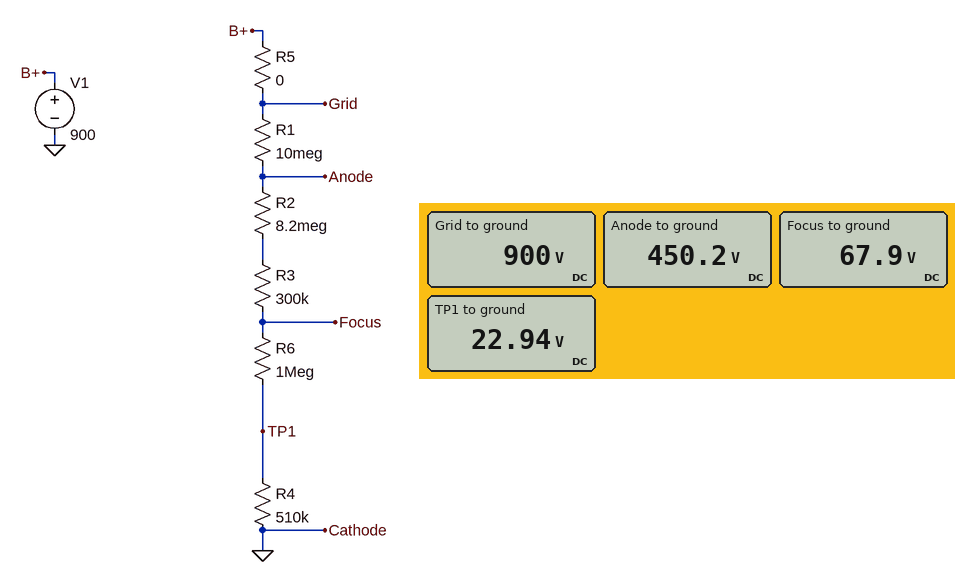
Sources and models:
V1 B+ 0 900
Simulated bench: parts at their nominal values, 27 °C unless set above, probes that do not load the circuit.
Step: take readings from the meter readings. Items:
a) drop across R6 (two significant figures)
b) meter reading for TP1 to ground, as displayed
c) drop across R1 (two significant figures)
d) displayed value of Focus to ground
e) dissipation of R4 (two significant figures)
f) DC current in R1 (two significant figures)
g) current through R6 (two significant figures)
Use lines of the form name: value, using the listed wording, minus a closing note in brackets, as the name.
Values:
drop across R6: 45 V
meter reading for TP1 to ground, as displayed: 22.94 V
drop across R1: 450 V
displayed value of Focus to ground: 67.9 V
dissipation of R4: 1.0 mW
DC current in R1: 45 µA
current through R6: 45 µA
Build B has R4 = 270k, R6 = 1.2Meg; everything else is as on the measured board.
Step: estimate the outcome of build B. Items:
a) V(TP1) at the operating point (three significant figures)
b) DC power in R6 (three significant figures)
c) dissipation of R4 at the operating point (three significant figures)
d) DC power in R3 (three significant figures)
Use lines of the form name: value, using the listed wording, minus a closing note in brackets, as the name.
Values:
V(TP1) at the operating point: 12.2 V
DC power in R6: 2.44 mW
dissipation of R4 at the operating point: 548 µW
DC power in R3: 609 µW
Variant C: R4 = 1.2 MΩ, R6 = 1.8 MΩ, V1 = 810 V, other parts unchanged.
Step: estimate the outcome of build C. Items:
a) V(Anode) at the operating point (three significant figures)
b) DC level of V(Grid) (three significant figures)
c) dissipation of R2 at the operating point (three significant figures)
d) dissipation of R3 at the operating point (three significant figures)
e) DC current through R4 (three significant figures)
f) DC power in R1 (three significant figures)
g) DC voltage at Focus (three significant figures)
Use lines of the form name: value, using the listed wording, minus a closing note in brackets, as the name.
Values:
V(Anode) at the operating point: 433 V
DC level of V(Grid): 810 V
dissipation of R2 at the operating point: 11.6 mW
dissipation of R3 at the operating point: 426 µW
DC current through R4: 37.7 µA
DC power in R1: 14.2 mW
DC voltage at Focus: 113 V
